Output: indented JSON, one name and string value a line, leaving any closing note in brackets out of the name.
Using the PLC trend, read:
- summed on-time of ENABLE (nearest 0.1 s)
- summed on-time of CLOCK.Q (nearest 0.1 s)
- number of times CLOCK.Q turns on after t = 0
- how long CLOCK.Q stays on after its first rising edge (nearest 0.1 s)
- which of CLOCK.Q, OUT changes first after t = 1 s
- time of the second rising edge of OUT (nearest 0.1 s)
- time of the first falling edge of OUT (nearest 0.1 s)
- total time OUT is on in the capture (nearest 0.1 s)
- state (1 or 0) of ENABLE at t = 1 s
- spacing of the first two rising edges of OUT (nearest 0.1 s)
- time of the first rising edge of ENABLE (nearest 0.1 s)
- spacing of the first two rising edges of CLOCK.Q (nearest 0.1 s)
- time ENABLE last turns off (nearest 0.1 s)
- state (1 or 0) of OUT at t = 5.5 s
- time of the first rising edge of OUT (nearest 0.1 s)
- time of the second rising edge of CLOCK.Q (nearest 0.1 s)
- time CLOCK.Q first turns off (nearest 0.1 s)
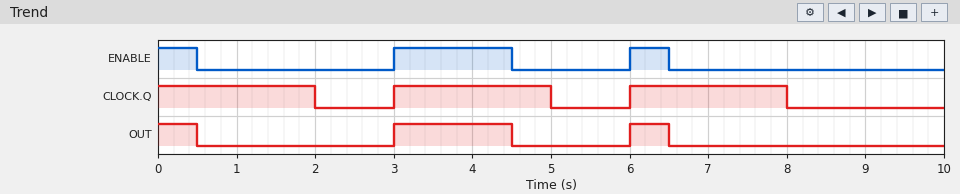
{
  "summed on-time of ENABLE": "2.5 s",
  "summed on-time of CLOCK.Q": "6.0 s",
  "number of times CLOCK.Q turns on after t = 0": "2",
  "how long CLOCK.Q stays on after its first rising edge": "2.0 s",
  "which of CLOCK.Q, OUT changes first after t = 1 s": "CLOCK.Q",
  "time of the second rising edge of OUT": "6.0 s",
  "time of the first falling edge of OUT": "0.5 s",
  "total time OUT is on in the capture": "2.5 s",
  "state (1 or 0) of ENABLE at t = 1 s": "0",
  "spacing of the first two rising edges of OUT": "3.0 s",
  "time of the first rising edge of ENABLE": "3.0 s",
  "spacing of the first two rising edges of CLOCK.Q": "3.0 s",
  "time ENABLE last turns off": "6.5 s",
  "state (1 or 0) of OUT at t = 5.5 s": "0",
  "time of the first rising edge of OUT": "3.0 s",
  "time of the second rising edge of CLOCK.Q": "6.0 s",
  "time CLOCK.Q first turns off": "2.0 s"
}
